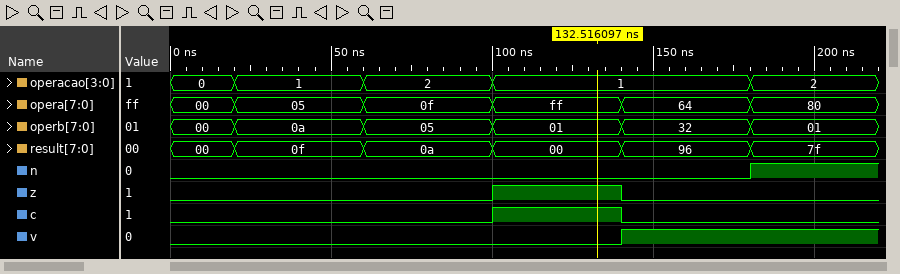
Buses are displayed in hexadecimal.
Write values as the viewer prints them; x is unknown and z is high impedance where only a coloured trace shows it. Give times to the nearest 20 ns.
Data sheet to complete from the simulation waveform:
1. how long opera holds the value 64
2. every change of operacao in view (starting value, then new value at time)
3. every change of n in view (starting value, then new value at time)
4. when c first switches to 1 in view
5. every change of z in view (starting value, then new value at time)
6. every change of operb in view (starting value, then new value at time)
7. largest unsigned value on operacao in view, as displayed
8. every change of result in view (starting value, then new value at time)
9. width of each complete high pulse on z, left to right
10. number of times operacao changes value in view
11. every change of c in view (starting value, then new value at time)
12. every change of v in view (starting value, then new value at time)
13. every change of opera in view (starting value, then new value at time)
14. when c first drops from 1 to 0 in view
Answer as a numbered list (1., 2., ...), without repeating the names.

1. 40 ns
2. 0, 1 at 20 ns, 2 at 60 ns, 1 at 100 ns, 2 at 180 ns
3. 0, 1 at 180 ns
4. 100 ns
5. 0, 1 at 100 ns, 0 at 140 ns
6. 00, 0a at 20 ns, 05 at 60 ns, 01 at 100 ns, 32 at 140 ns, 01 at 180 ns
7. 2
8. 00, 0f at 20 ns, 0a at 60 ns, 00 at 100 ns, 96 at 140 ns, 7f at 180 ns
9. 40 ns
10. 4
11. 0, 1 at 100 ns, 0 at 140 ns
12. 0, 1 at 140 ns
13. 00, 05 at 20 ns, 0f at 60 ns, ff at 100 ns, 64 at 140 ns, 80 at 180 ns
14. 140 ns
